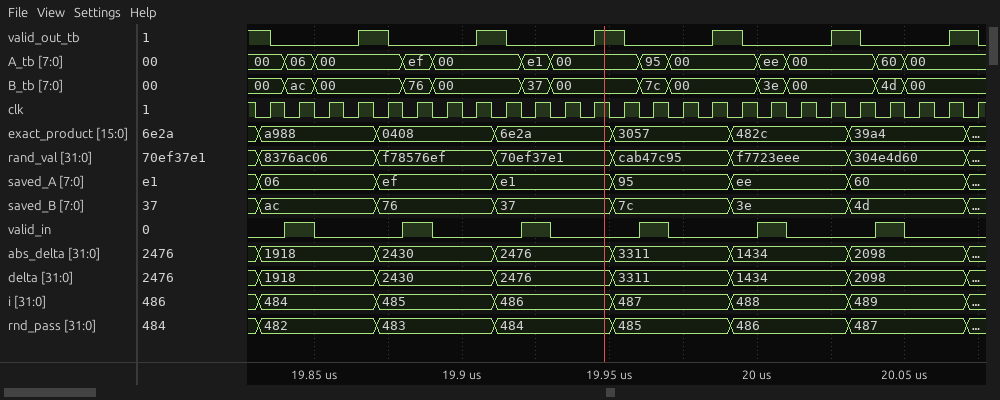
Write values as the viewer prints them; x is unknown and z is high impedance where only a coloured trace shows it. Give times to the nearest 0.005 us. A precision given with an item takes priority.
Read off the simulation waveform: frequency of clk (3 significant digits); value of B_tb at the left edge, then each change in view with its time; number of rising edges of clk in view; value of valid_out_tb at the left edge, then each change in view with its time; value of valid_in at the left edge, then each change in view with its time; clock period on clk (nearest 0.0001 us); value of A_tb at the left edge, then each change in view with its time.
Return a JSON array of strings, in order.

["100 MHz", "00, ac at 19.84 us, 00 at 19.85 us, 76 at 19.88 us, 00 at 19.89 us, 37 at 19.92 us, 00 at 19.93 us, 7c at 19.96 us, 00 at 19.97 us, 3e at 20 us, 00 at 20.01 us, 4d at 20.04 us, 00 at 20.05 us", "25", "1, 0 at 19.835 us, 1 at 19.865 us, 0 at 19.875 us, 1 at 19.905 us, 0 at 19.915 us, 1 at 19.945 us, 0 at 19.955 us, 1 at 19.985 us, 0 at 19.995 us, 1 at 20.025 us, 0 at 20.035 us, 1 at 20.065 us, 0 at 20.075 us", "0, 1 at 19.84 us, 0 at 19.85 us, 1 at 19.88 us, 0 at 19.89 us, 1 at 19.92 us, 0 at 19.93 us, 1 at 19.96 us, 0 at 19.97 us, 1 at 20 us, 0 at 20.01 us, 1 at 20.04 us, 0 at 20.05 us", "0.01 us", "00, 06 at 19.84 us, 00 at 19.85 us, ef at 19.88 us, 00 at 19.89 us, e1 at 19.92 us, 00 at 19.93 us, 95 at 19.96 us, 00 at 19.97 us, ee at 20 us, 00 at 20.01 us, 60 at 20.04 us, 00 at 20.05 us"]
